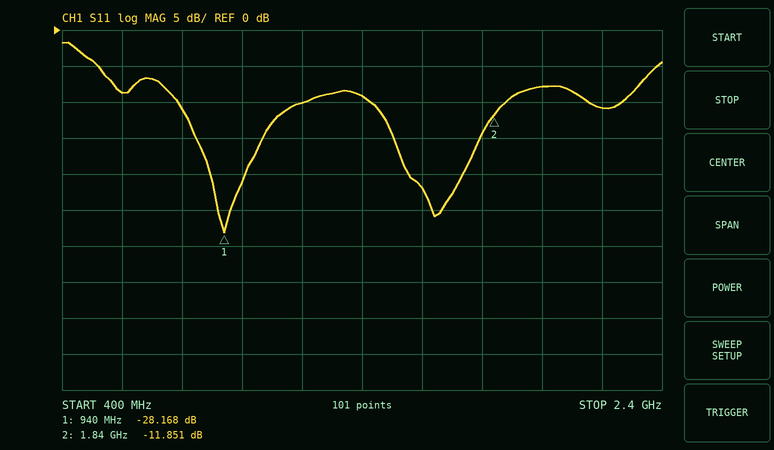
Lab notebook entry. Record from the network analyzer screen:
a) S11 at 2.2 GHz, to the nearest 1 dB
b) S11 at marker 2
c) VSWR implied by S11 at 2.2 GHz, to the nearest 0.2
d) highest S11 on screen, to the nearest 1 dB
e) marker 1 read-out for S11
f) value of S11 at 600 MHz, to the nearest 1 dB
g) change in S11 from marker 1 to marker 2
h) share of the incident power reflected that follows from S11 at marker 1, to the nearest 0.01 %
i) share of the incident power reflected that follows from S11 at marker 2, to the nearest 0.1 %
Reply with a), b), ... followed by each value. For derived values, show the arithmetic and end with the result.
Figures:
a) -11 dB
b) -11.851 dB
c) |Γ| = 10^(-11/20) = 0.2818; VSWR = (1 + 0.2818)/(1 − 0.2818) ≈ 1.8
d) -2 dB
e) -28.168 dB
f) -9 dB
g) -11.851 − (-28.168) = 16.317 dB
h) 10^(-28.168/10) ≈ 0.15 %
i) 10^(-11.851/10) ≈ 6.5 %
